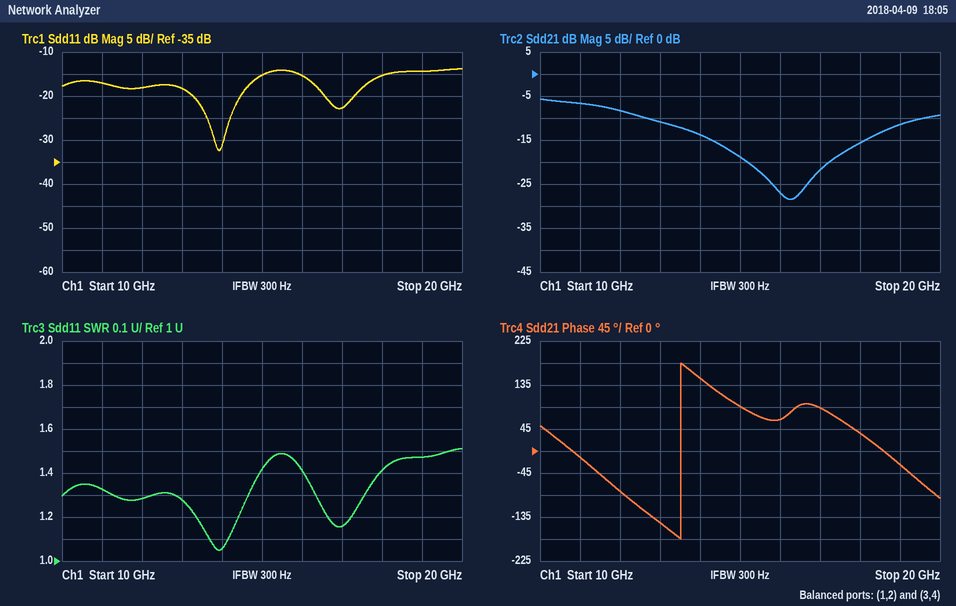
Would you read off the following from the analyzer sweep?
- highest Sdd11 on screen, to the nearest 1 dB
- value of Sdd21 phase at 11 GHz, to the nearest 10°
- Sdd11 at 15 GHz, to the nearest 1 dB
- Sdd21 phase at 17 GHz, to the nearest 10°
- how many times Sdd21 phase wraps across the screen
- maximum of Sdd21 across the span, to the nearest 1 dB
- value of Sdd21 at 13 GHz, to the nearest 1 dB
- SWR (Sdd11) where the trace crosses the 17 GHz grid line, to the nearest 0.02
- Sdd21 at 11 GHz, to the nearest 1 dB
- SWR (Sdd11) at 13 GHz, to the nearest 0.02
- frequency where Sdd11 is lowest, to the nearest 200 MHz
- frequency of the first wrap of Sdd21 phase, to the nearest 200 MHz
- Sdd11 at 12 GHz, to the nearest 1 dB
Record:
-14 dB
-10°
-15 dB
90°
1
-6 dB
-11 dB
1.16
-7 dB
1.28
14.0 GHz
13.6 GHz
-18 dB
